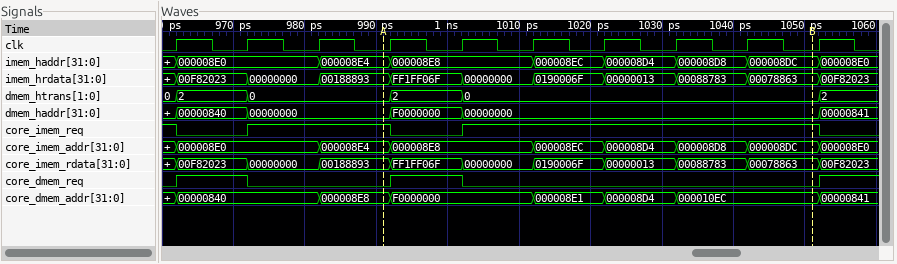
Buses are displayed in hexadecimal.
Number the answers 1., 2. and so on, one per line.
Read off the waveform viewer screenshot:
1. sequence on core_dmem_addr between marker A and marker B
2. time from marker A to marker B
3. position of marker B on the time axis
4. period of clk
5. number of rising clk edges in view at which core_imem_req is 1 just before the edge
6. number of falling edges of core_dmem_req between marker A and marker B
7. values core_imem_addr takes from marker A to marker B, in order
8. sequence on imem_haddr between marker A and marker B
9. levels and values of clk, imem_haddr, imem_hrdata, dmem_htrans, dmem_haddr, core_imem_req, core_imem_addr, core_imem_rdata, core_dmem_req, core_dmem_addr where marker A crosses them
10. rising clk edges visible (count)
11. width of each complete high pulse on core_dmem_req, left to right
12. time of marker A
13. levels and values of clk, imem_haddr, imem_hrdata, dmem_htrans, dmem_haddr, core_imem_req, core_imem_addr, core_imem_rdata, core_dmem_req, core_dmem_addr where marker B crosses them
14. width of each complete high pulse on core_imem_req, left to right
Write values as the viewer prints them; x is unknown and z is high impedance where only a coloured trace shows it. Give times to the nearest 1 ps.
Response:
1. 000008E8, F0000000, 000008E1, 000008D4, 000010EC
2. 60 ps
3. 1051 ps
4. 10 ps
5. 8
6. 1
7. 000008E4, 000008E8, 000008EC, 000008D4, 000008D8, 000008DC
8. 000008E4, 000008E8, 000008EC, 000008D4, 000008D8, 000008DC
9. clk=0, imem_haddr=000008E4, imem_hrdata=00188893, dmem_htrans=0, dmem_haddr=00000000, core_imem_req=1, core_imem_addr=000008E4, core_imem_rdata=00188893, core_dmem_req=0, core_dmem_addr=000008E8
10. 10
11. 10 ps, 10 ps
12. 991 ps
13. clk=0, imem_haddr=000008DC, imem_hrdata=00078863, dmem_htrans=0, dmem_haddr=00000000, core_imem_req=1, core_imem_addr=000008DC, core_imem_rdata=00078863, core_dmem_req=0, core_dmem_addr=000010EC
14. 20 ps, 50 ps
